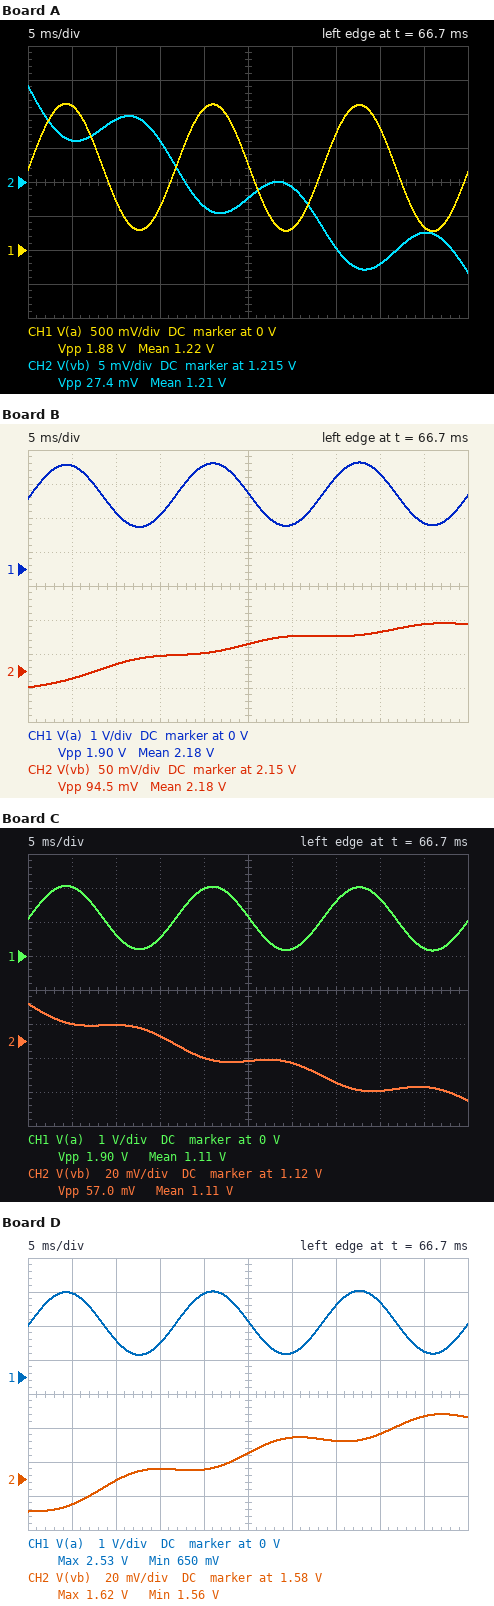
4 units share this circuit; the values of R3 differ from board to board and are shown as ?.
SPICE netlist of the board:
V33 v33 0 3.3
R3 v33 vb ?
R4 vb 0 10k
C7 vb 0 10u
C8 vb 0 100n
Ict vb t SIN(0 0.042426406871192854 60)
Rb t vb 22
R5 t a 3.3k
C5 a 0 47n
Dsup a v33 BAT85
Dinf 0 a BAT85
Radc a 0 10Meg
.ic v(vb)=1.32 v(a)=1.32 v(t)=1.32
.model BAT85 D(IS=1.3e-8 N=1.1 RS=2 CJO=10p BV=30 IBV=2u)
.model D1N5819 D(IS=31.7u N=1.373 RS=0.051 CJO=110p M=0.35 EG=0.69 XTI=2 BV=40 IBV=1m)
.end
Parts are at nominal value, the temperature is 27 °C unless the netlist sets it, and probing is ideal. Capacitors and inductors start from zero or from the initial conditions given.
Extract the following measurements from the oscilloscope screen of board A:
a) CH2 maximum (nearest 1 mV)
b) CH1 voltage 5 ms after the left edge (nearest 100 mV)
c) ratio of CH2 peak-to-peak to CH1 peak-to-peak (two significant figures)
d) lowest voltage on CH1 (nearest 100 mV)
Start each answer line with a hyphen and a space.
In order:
- 1.229 V
- 2.1 V
- 0.015
- 300 mV
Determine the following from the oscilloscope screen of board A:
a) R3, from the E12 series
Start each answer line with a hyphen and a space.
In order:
- 18 kΩ
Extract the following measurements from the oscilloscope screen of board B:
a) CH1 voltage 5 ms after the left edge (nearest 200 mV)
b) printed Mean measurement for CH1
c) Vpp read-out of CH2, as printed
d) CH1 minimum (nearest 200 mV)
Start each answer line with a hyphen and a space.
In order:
- 3.0 V
- 2.18 V
- 94.5 mV
- 1.2 V
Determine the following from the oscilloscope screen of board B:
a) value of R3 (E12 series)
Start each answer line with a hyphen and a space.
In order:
- 4.7 kΩ
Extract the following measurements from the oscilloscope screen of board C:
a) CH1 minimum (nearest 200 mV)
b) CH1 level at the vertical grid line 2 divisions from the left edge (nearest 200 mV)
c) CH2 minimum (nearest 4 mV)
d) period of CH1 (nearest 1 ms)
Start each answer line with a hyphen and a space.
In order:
- 200 mV
- 600 mV
- 1.084 V
- 17 ms
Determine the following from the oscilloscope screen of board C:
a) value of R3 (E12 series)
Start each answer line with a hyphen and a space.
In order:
- 22 kΩ
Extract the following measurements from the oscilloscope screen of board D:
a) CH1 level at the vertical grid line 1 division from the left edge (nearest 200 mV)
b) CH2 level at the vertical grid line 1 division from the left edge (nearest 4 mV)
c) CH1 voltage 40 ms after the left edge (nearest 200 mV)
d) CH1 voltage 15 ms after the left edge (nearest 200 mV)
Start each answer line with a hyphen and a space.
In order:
- 2.4 V
- 1.564 V
- 2.2 V
- 1.0 V
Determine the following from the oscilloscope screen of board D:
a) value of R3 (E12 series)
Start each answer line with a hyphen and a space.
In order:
- 10 kΩ
